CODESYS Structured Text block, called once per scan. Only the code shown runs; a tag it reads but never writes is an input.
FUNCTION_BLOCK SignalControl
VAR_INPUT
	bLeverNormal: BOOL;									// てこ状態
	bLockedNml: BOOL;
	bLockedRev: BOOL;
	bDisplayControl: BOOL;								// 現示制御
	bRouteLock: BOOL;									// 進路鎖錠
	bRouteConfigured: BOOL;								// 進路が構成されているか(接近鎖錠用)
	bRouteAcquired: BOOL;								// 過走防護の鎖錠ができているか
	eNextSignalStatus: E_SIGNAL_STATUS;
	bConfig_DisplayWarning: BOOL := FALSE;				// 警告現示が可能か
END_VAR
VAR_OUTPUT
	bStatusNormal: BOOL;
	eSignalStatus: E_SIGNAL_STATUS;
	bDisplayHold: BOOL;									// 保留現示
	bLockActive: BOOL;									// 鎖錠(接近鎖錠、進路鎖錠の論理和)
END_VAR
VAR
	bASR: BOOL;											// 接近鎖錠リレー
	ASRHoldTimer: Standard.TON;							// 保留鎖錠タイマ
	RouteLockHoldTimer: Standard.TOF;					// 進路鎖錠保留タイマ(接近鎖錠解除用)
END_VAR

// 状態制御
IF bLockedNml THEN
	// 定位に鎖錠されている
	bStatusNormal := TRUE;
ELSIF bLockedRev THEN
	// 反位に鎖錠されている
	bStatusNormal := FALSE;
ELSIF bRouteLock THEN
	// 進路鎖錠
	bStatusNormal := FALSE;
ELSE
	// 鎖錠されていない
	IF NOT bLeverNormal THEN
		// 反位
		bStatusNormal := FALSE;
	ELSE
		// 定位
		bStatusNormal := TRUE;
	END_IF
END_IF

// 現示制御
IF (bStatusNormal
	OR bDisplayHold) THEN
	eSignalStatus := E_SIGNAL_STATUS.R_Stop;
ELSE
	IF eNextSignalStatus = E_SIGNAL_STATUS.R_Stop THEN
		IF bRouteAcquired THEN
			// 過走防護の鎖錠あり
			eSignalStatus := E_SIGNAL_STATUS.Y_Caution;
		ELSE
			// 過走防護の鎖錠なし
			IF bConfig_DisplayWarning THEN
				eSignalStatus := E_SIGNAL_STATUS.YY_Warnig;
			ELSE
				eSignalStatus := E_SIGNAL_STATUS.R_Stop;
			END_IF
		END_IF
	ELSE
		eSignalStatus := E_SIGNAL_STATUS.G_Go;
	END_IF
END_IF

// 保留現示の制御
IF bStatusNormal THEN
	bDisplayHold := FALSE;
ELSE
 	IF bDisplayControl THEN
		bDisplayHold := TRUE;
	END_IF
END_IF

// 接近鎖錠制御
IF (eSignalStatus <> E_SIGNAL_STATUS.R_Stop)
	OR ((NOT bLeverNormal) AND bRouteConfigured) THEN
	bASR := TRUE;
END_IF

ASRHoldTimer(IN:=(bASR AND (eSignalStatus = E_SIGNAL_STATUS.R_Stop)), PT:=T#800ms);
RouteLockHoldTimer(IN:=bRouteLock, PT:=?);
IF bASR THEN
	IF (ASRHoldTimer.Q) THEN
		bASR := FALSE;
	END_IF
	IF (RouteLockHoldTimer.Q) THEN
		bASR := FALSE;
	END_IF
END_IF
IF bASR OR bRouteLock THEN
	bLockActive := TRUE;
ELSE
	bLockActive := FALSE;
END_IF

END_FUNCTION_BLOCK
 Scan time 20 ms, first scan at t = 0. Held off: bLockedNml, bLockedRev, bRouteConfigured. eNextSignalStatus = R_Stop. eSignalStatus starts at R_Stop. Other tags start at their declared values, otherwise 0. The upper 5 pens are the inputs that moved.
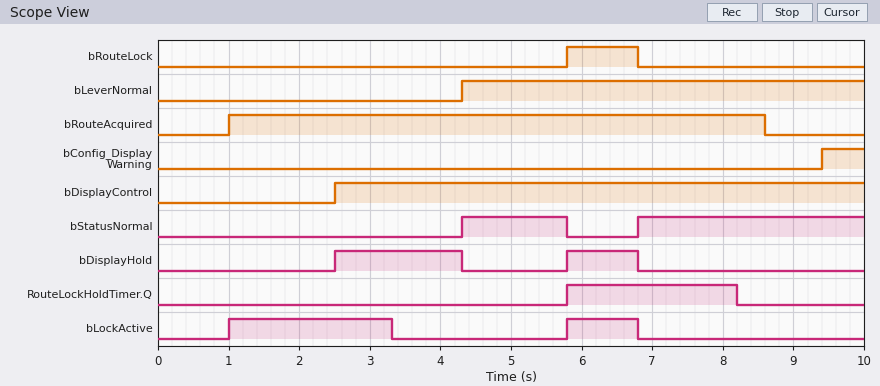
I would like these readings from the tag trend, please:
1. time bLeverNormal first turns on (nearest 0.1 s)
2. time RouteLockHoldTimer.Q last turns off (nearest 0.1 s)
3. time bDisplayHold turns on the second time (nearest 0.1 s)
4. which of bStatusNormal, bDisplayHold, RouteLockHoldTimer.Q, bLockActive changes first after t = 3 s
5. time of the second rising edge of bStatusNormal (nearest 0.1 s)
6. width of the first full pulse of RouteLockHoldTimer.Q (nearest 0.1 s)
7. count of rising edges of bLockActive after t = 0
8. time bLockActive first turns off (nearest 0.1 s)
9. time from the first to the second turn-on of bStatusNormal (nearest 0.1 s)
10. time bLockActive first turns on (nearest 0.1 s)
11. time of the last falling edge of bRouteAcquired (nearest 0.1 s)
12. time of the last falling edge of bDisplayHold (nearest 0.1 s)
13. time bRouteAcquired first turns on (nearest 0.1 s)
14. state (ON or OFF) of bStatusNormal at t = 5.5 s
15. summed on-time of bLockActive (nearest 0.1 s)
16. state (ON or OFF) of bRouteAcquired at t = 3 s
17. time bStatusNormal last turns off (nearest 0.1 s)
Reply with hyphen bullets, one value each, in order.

- 4.3 s
- 8.2 s
- 5.8 s
- bLockActive
- 6.8 s
- 2.4 s
- 2
- 3.3 s
- 2.5 s
- 1.0 s
- 8.6 s
- 6.8 s
- 1.0 s
- ON
- 3.3 s
- ON
- 5.8 s
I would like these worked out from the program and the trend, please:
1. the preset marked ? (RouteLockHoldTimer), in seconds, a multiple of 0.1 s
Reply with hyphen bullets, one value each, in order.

- 1.4 s
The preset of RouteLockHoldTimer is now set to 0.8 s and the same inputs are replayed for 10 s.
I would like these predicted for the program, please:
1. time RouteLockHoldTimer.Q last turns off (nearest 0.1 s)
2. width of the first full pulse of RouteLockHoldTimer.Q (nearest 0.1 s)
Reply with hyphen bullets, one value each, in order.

- 7.6 s
- 1.8 s
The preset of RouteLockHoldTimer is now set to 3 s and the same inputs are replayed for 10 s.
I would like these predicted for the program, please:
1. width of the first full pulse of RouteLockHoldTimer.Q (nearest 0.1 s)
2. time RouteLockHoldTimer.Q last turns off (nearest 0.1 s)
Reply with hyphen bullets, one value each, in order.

- 4.0 s
- 9.8 s
